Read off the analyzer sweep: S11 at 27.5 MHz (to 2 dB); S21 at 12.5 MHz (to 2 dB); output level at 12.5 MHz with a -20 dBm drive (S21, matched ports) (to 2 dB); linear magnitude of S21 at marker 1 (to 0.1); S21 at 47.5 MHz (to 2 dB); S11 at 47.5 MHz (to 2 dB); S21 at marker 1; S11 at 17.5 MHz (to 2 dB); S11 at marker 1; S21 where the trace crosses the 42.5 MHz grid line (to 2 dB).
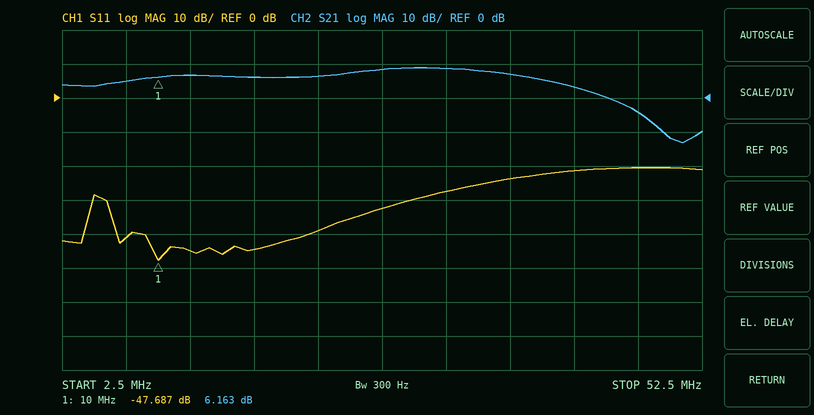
-32 dB
6 dB
-14 dBm
2.0
-4 dB
-20 dB
6.163 dB
-44 dB
-47.687 dB
4 dB
